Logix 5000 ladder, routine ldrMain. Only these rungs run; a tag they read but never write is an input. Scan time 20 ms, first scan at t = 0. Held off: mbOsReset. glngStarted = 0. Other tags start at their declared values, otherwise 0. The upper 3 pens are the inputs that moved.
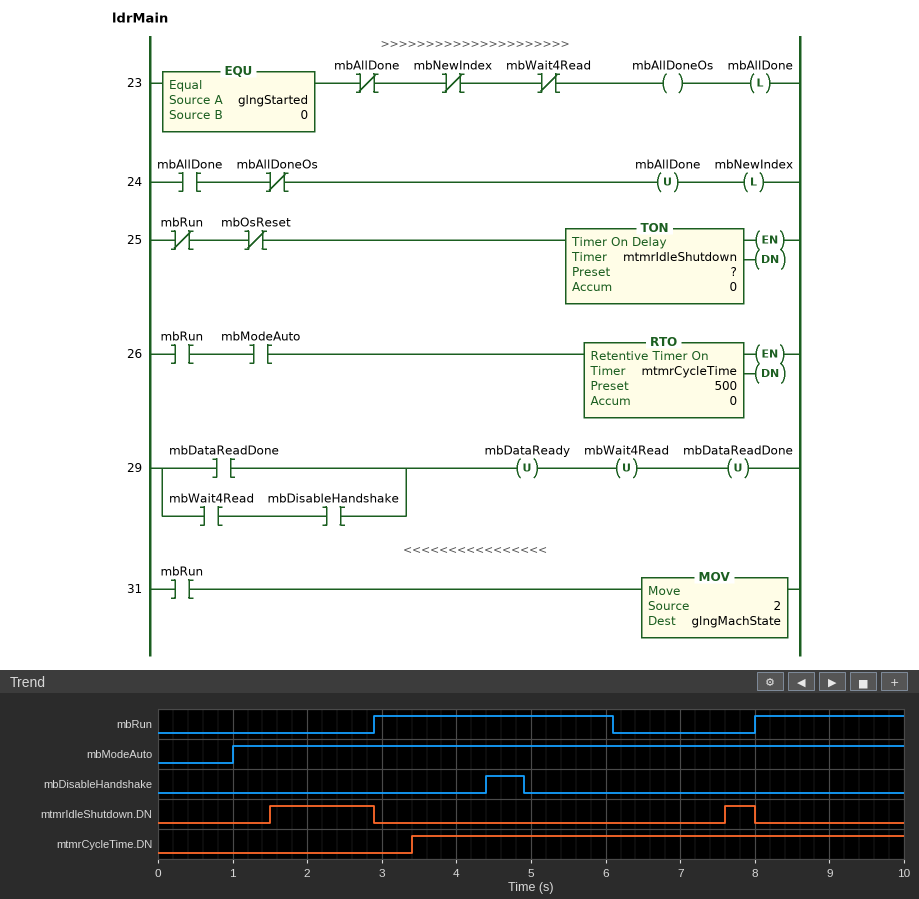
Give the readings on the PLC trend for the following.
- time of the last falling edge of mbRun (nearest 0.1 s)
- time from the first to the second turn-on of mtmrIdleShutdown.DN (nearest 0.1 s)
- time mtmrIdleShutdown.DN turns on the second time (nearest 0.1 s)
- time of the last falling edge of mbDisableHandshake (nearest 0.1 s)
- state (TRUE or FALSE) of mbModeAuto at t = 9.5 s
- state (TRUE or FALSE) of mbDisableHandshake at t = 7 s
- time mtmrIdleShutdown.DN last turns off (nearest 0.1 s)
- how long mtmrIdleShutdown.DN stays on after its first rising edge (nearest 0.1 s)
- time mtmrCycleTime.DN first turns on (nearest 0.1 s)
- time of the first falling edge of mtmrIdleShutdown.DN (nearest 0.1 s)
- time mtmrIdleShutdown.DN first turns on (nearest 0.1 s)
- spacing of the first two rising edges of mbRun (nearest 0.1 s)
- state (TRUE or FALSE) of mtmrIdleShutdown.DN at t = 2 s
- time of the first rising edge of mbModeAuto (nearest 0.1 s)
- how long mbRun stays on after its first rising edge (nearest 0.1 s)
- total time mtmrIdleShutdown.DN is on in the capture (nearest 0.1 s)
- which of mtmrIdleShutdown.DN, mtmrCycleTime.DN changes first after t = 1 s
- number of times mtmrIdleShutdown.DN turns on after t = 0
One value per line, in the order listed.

6.1 s
6.1 s
7.6 s
4.9 s
TRUE
FALSE
8.0 s
1.4 s
3.4 s
2.9 s
1.5 s
5.1 s
TRUE
1.0 s
3.2 s
1.8 s
mtmrIdleShutdown.DN
2
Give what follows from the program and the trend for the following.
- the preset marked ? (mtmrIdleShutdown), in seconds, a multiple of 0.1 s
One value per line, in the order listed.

1.5 s
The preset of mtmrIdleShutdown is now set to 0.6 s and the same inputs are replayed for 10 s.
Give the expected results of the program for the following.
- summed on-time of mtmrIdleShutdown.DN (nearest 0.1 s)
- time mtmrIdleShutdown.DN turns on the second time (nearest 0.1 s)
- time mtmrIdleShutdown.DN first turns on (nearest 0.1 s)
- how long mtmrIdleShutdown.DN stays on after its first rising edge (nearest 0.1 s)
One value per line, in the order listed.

3.6 s
6.7 s
0.6 s
2.3 s
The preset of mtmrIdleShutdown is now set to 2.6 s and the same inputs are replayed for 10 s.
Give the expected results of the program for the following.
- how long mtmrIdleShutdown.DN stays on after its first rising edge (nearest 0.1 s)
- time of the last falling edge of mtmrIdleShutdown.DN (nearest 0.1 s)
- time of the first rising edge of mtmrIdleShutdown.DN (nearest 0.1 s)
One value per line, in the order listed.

0.3 s
2.9 s
2.6 s
